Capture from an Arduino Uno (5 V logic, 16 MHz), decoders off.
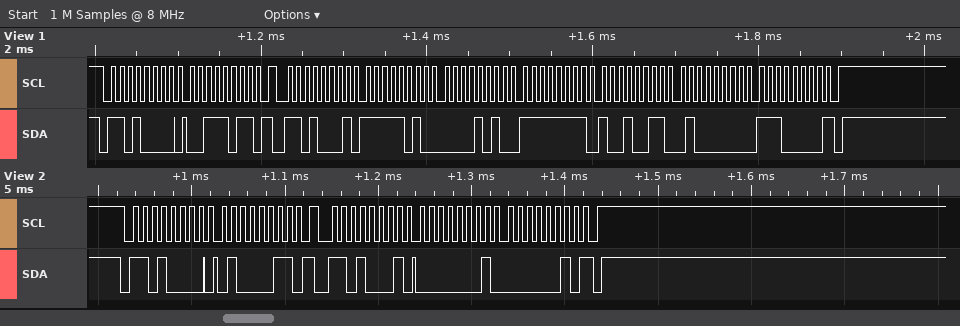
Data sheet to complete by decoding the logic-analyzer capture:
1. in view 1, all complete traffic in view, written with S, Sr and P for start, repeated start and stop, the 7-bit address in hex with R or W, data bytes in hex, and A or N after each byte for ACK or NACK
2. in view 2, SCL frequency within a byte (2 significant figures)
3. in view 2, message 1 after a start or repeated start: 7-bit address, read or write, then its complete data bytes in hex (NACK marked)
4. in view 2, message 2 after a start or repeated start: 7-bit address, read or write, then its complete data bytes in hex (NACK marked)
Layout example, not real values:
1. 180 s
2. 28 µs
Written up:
1. S 68W A 3B A Sr 68R A FA A 0A A FF A 93 A 40 A E0 N P
2. 100 kHz
3. 0x68 write: 43
4. 0x68 read: 01 02 NACK
